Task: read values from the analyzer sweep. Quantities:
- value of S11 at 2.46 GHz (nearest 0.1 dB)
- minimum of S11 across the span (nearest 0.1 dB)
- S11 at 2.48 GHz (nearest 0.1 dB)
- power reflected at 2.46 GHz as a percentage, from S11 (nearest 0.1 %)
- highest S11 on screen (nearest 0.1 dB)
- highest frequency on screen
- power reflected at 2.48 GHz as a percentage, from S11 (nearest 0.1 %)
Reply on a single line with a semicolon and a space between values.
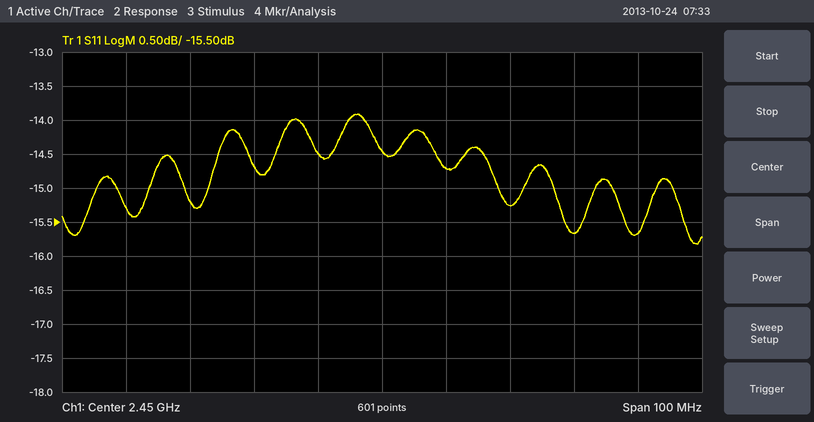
-14.7 dB; -15.8 dB; -15.7 dB; 3.4 %; -13.9 dB; 2.5 GHz; 2.7 %
